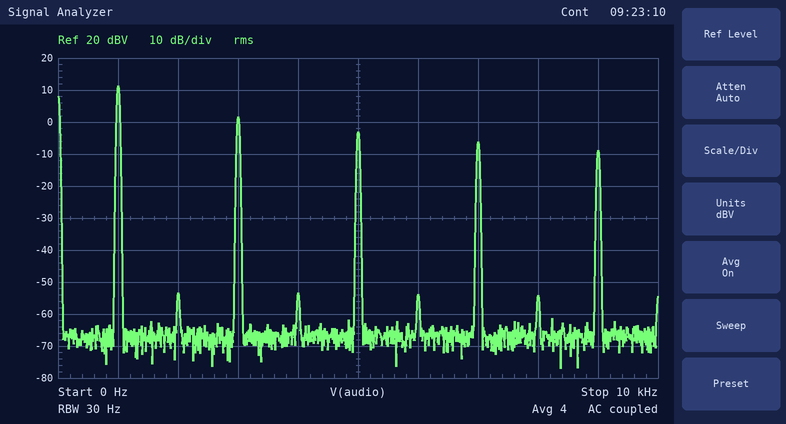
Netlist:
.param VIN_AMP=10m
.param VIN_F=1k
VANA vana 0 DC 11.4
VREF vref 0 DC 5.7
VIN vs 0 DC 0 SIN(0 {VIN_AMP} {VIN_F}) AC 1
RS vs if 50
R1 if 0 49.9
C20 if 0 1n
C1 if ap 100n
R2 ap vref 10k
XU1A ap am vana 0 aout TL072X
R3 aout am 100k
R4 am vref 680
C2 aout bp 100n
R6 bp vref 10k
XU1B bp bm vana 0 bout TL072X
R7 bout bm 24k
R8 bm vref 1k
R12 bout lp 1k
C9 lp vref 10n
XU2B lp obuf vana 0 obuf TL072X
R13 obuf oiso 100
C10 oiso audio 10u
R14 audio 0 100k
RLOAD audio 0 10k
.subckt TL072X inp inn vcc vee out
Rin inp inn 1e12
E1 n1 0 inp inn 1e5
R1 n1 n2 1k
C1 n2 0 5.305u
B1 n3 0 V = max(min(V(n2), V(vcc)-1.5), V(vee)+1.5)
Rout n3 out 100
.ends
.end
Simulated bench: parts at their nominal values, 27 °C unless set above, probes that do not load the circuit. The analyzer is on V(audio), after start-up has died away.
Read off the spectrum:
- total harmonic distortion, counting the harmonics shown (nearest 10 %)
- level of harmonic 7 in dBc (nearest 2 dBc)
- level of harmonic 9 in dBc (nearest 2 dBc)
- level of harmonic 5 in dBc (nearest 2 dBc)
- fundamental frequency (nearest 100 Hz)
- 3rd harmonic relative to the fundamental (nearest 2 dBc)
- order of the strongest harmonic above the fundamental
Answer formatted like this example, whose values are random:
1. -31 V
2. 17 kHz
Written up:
1. 40 %
2. -18 dBc
3. -20 dBc
4. -14 dBc
5. 1.0 kHz
6. -10 dBc
7. 3
